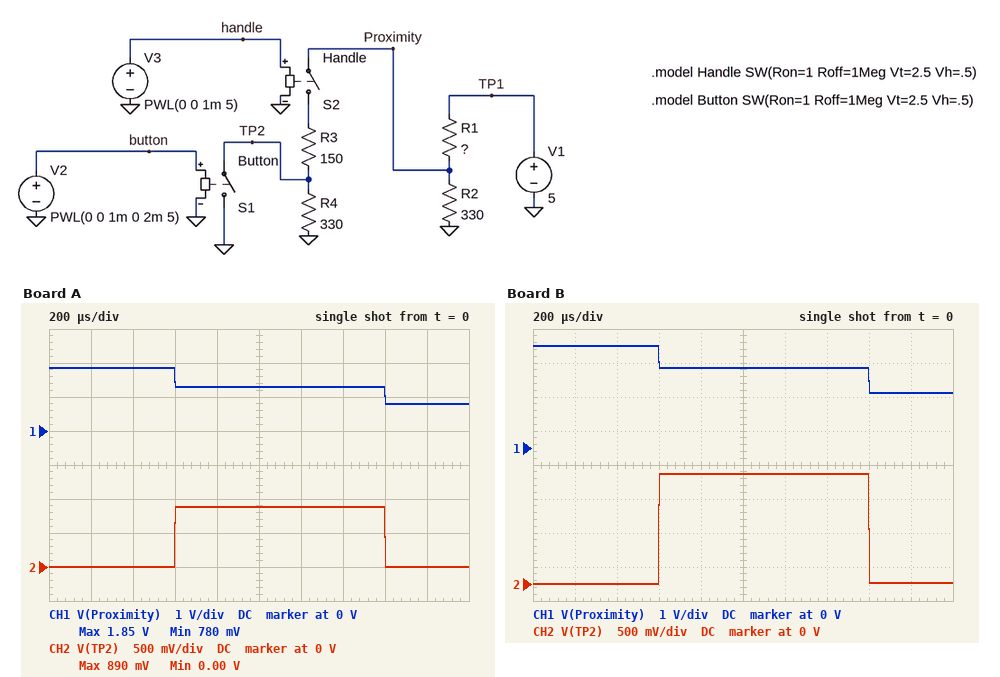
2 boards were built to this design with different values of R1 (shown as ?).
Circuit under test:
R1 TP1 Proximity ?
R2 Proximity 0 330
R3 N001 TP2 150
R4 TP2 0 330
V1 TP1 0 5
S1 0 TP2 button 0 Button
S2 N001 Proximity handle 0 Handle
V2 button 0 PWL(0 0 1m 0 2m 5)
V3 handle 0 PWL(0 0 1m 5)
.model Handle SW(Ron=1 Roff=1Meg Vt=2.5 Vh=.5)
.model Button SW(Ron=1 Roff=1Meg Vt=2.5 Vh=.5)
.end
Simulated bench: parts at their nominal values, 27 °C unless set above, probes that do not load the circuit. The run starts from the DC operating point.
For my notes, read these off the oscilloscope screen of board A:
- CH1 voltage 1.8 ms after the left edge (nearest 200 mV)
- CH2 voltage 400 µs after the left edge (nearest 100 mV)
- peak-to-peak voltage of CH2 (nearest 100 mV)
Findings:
800 mV
0 V
900 mV
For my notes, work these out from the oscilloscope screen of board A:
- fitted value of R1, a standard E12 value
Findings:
560 Ω
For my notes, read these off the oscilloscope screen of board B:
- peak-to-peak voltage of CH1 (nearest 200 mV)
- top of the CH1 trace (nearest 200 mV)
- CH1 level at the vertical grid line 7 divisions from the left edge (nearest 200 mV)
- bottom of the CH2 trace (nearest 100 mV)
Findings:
1.4 V
3.0 V
2.4 V
0 V
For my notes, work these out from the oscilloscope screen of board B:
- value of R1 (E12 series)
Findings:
220 Ω
